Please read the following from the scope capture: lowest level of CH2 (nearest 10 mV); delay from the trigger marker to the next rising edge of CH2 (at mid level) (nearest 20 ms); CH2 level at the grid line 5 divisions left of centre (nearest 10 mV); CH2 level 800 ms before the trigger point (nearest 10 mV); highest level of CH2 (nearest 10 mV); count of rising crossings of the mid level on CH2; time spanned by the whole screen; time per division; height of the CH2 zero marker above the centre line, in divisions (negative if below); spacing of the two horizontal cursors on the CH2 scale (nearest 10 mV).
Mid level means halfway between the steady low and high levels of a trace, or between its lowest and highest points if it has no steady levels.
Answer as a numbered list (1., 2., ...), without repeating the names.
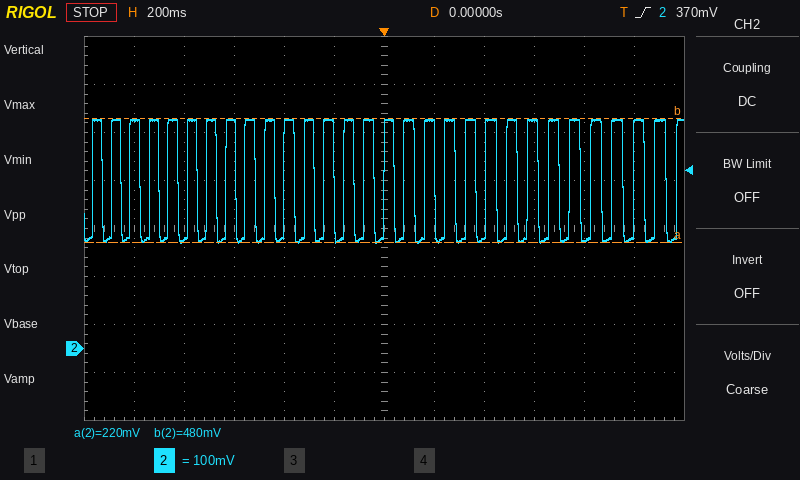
1. 220 mV
2. 80 ms
3. 480 mV
4. 230 mV
5. 480 mV
6. 30
7. 2.4 s
8. 200 ms
9. -2.5 div
10. 260 mV
